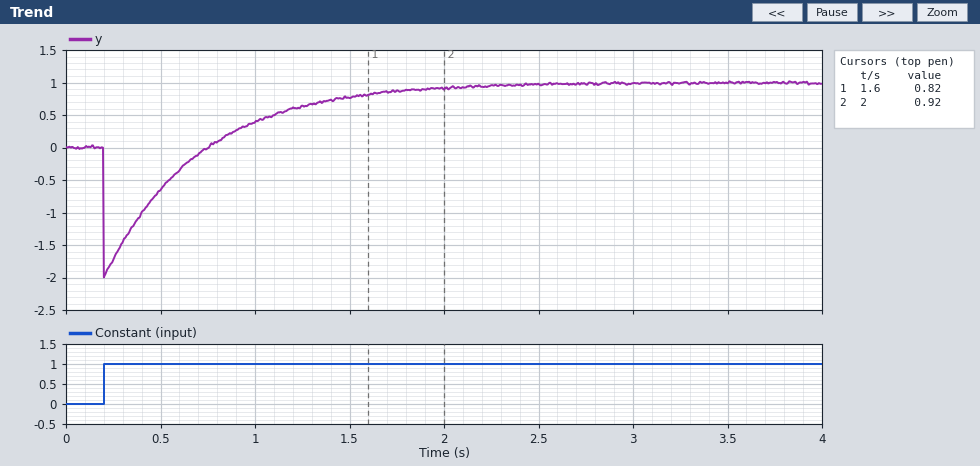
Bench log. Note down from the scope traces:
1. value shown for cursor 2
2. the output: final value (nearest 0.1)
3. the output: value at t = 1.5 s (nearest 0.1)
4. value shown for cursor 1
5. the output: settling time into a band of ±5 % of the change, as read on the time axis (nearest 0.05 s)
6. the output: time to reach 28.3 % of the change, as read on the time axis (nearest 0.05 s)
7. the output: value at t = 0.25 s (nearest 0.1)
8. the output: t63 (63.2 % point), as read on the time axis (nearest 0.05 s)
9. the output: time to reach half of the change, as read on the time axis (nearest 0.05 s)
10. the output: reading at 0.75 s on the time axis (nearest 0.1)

0.92
1.0
0.8
0.82
2.25 s
0.90 s
-1.7
1.25 s
1.10 s
0.0
